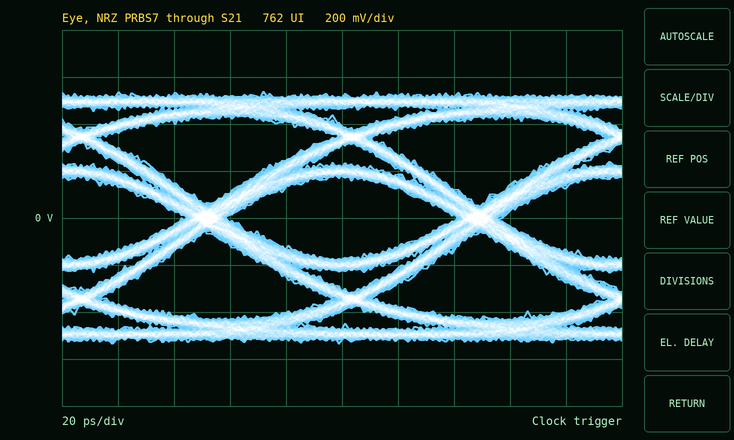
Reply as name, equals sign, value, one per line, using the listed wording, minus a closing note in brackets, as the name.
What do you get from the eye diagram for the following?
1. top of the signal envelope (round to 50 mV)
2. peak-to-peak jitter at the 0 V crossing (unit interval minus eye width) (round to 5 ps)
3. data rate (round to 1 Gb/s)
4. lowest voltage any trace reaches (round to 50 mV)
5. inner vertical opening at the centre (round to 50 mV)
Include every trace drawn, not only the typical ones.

top of the signal envelope = 550 mV
peak-to-peak jitter at the 0 V crossing (unit interval minus eye width) = 15 ps
data rate = 10 Gb/s
lowest voltage any trace reaches = -550 mV
inner vertical opening at the centre = 350 mV
